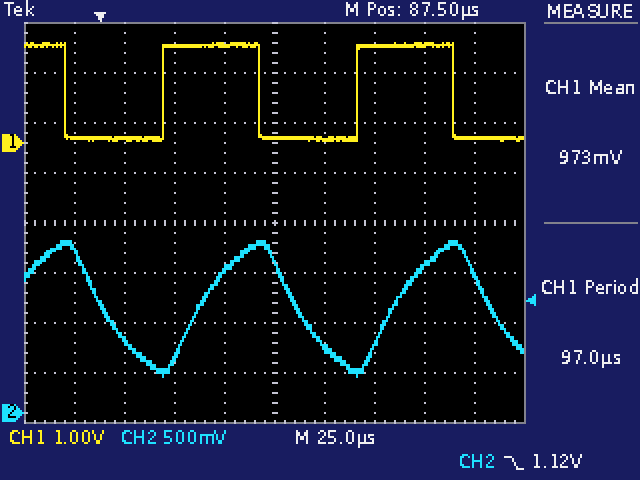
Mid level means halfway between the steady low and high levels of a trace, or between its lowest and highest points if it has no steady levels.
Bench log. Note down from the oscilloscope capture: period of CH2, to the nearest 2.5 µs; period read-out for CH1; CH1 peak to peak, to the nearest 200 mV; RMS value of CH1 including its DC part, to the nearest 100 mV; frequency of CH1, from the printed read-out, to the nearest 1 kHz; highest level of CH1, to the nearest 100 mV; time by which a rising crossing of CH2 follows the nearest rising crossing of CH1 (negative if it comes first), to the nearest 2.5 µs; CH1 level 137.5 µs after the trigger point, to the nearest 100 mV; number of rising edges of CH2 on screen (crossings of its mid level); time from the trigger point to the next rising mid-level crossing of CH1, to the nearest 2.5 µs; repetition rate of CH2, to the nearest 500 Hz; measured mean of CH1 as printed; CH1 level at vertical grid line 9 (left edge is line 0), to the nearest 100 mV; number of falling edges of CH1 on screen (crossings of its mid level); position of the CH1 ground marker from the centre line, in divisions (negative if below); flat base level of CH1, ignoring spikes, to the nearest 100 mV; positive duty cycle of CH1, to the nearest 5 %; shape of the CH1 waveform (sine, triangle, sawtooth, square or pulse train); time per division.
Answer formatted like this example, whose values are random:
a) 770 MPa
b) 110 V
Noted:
a) 97.5 µs
b) 97.0 µs
c) 2.0 V
d) 1.4 V
e) 10 kHz
f) 2.0 V
g) +17.5 µs
h) 1.9 V
i) 2
j) 32.5 µs
k) 10.5 kHz
l) 973 mV
m) 100 mV
n) 3
o) +1.6 div
p) 100 mV
q) 50 %
r) square
s) 25 µs
